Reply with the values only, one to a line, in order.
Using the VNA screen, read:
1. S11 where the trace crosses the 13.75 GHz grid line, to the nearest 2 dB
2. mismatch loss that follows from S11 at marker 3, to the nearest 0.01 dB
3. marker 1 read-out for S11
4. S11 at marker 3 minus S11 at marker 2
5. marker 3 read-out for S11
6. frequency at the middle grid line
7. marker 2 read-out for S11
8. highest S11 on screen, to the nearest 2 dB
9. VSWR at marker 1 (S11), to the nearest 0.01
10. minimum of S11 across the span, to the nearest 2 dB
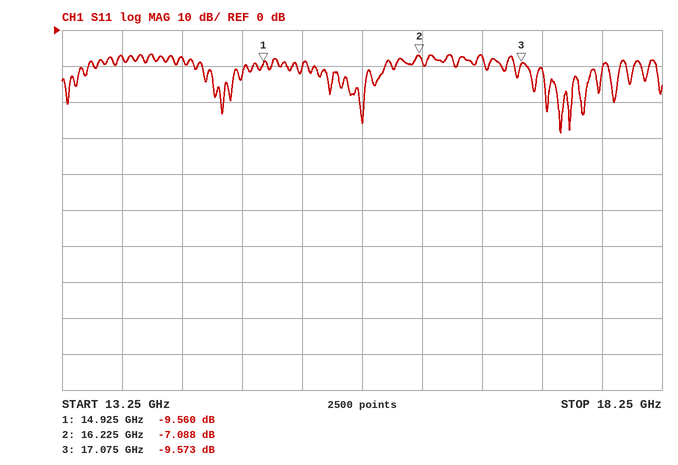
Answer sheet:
-8 dB
0.51 dB
-9.560 dB
-2.485 dB
-9.573 dB
15.75 GHz
-7.088 dB
-6 dB
2.00
-28 dB
